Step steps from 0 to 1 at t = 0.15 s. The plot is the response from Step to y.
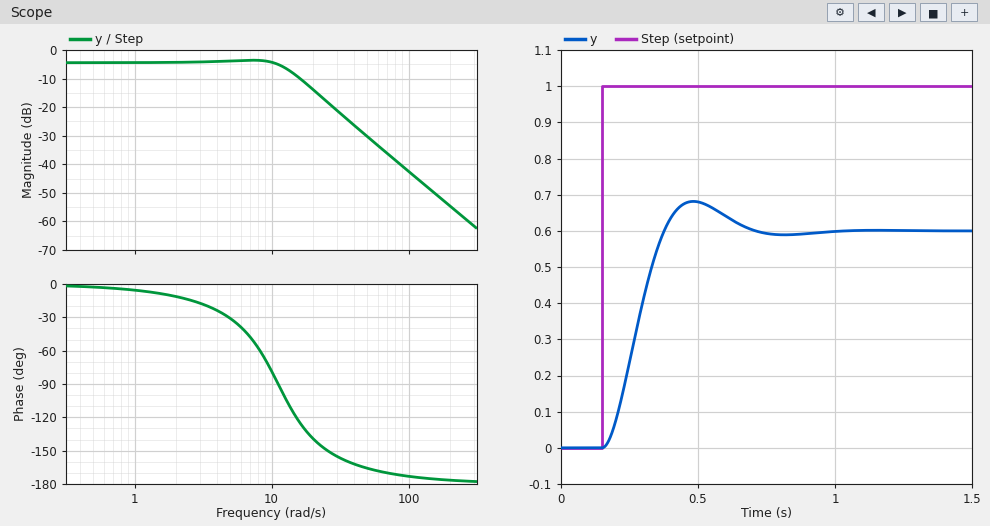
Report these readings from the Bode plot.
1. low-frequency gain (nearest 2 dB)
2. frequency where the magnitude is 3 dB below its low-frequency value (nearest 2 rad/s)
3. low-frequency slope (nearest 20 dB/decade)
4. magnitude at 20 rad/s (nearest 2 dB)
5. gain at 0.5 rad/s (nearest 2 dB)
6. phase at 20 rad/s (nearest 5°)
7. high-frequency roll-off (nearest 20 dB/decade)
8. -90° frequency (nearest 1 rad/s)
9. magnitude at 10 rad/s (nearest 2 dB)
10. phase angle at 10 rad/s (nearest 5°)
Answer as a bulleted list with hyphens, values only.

- -4 dB
- 14 rad/s
- 0 dB/decade
- -14 dB
- -4 dB
- -140°
- -40 dB/decade
- 11 rad/s
- -4 dB
- -80°
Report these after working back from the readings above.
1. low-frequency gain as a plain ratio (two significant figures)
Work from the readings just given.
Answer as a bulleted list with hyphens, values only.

- 0.63
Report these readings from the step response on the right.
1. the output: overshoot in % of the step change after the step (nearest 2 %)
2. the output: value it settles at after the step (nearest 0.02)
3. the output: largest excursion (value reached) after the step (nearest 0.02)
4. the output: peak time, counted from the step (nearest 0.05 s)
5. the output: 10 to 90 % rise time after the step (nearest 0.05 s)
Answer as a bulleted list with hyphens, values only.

- 14 %
- 0.60
- 0.68
- 0.35 s
- 0.15 s
